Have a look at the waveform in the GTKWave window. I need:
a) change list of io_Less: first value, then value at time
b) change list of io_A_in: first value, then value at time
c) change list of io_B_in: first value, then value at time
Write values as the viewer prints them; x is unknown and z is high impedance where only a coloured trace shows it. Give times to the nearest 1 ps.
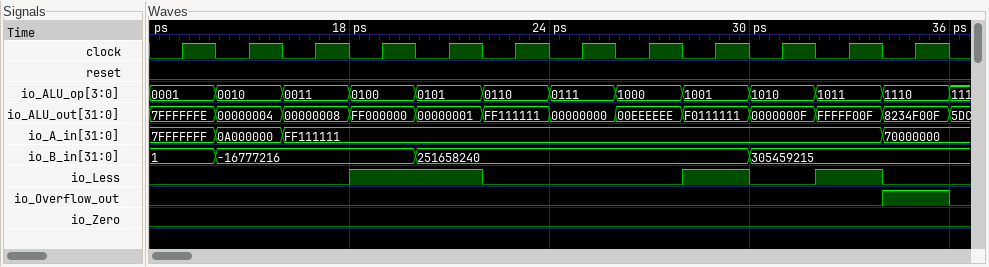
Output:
0, 1 at 18 ps, 0 at 22 ps, 1 at 28 ps, 0 at 30 ps, 1 at 32 ps, 0 at 34 ps
7FFFFFFF, 0A000000 at 14 ps, FF111111 at 16 ps, 70000000 at 34 ps
1, -16777216 at 14 ps, 251658240 at 20 ps, 305459215 at 30 ps
